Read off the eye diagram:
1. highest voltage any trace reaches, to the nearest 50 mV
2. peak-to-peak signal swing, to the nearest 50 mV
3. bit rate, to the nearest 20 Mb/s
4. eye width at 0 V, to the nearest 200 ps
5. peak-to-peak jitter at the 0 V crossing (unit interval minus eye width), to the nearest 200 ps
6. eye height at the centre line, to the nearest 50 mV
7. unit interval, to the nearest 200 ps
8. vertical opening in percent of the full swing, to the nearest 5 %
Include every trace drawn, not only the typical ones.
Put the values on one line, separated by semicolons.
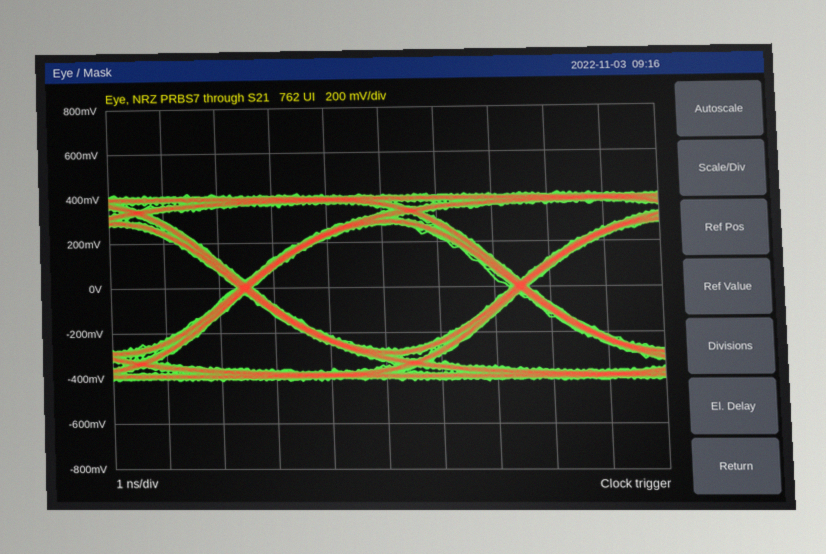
400 mV; 850 mV; 200 Mb/s; 4.6 ns; 400 ps; 550 mV; 5.0 ns; 65 %
